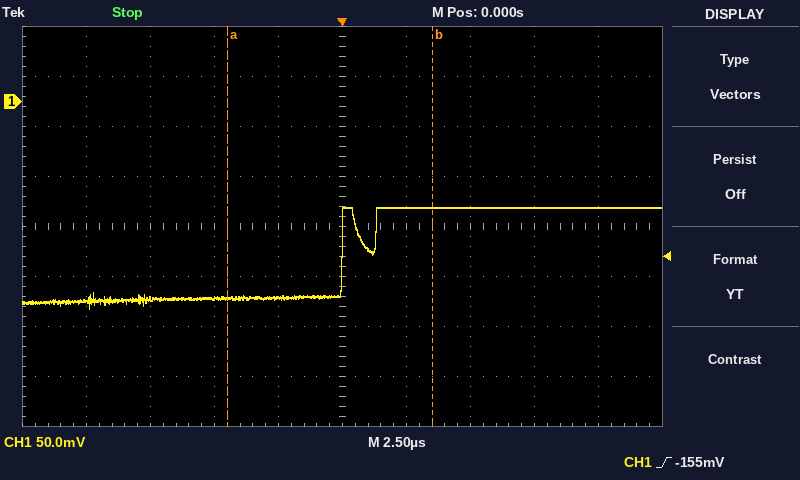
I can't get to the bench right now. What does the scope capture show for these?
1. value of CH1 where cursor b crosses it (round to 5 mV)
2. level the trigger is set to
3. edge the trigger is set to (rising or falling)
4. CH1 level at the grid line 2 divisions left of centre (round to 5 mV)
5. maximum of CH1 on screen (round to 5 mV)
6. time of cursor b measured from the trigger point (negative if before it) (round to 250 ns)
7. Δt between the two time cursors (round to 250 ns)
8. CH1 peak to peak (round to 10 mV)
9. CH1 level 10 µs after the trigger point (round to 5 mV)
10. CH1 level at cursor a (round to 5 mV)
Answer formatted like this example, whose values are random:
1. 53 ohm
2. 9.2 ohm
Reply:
1. -105 mV
2. -155 mV
3. rising
4. -195 mV
5. -105 mV
6. +3.50 µs
7. 8.00 µs
8. 100 mV
9. -105 mV
10. -195 mV
